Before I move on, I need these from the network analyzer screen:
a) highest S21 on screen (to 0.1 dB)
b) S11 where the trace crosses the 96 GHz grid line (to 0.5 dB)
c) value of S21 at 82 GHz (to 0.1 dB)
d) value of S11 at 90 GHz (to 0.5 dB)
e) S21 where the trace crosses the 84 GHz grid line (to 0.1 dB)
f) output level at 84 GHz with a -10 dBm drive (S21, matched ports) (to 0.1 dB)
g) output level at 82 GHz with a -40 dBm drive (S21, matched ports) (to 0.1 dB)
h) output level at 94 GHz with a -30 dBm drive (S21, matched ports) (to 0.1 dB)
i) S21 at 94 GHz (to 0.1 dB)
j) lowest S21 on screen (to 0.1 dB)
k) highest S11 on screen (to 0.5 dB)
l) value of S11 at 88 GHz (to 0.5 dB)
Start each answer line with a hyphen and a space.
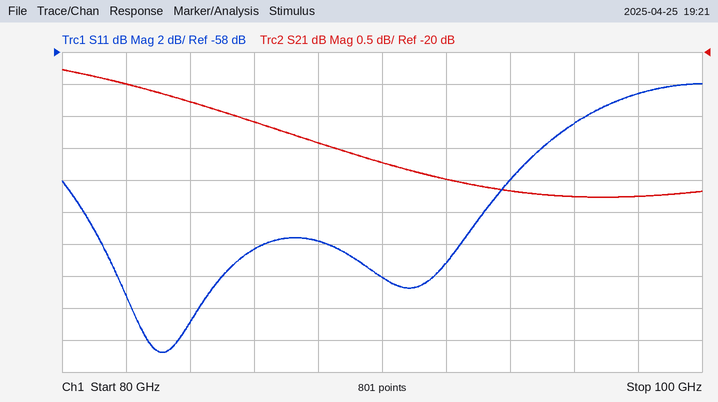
- -20.3 dB
- -62.5 dB
- -20.5 dB
- -72.0 dB
- -20.8 dB
- -30.8 dBm
- -60.5 dBm
- -52.2 dBm
- -22.2 dB
- -22.3 dB
- -60.0 dB
- -70.0 dB
